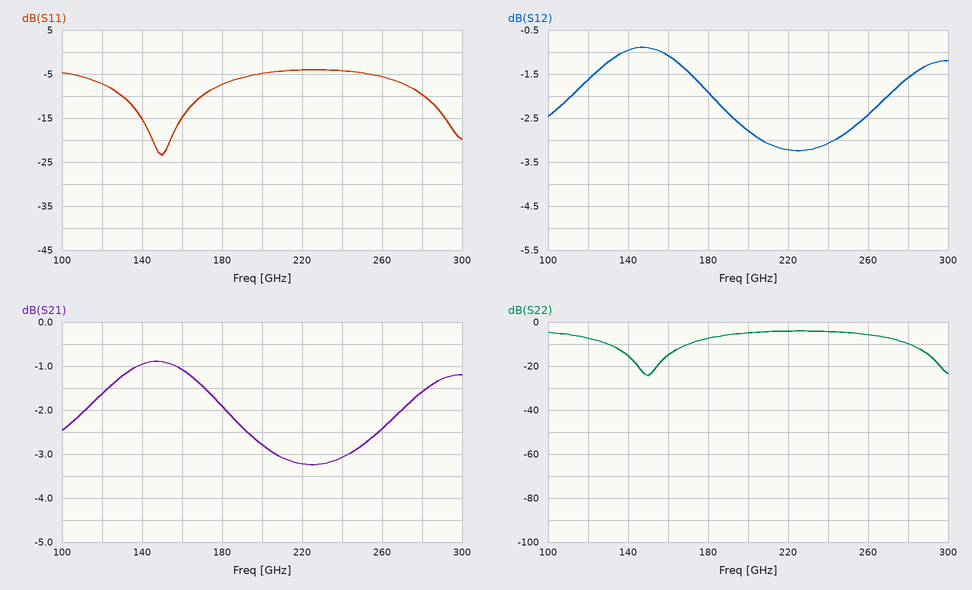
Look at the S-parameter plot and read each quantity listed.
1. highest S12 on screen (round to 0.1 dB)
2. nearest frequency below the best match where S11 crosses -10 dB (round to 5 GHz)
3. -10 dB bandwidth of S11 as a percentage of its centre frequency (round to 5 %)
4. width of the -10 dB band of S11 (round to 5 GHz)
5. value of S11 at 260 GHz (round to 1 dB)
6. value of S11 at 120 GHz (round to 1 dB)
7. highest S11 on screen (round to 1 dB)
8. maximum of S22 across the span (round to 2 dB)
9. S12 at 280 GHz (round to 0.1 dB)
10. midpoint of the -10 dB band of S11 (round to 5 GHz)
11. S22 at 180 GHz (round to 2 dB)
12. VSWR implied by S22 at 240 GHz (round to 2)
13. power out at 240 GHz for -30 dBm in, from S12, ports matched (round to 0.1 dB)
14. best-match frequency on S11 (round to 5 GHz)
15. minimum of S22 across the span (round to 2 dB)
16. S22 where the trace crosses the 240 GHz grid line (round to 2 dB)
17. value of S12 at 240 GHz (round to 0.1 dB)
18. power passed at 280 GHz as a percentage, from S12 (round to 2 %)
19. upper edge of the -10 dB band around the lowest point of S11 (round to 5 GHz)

-0.9 dB
130 GHz
25 %
40 GHz
-6 dB
-7 dB
-4 dB
-4 dB
-1.6 dB
150 GHz
-8 dB
4
-33.1 dBm
150 GHz
-24 dB
-4 dB
-3.1 dB
70 %
170 GHz
